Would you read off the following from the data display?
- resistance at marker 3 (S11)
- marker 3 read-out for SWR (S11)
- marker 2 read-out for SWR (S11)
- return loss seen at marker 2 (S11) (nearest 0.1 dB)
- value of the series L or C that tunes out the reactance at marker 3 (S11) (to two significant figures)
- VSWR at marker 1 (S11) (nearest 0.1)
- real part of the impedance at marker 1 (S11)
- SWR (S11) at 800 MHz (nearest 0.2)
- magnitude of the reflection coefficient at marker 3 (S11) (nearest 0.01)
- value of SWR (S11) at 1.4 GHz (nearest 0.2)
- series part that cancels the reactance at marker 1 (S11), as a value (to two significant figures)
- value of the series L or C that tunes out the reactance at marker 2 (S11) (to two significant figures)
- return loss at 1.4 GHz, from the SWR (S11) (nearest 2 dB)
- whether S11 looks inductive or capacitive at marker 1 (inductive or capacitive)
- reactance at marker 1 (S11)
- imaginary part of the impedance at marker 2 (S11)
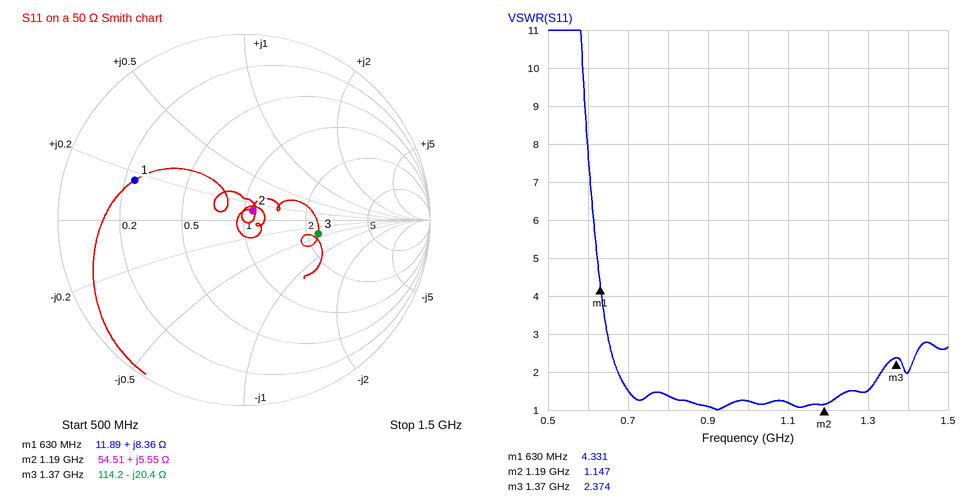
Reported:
114.2 Ω
2.374
1.147
23.3 dB
2.4 nH
4.3
11.89 Ω
1.4
0.41
2.0
30 pF
24 pF
10 dB
inductive
+8.36 Ω
+5.55 Ω
